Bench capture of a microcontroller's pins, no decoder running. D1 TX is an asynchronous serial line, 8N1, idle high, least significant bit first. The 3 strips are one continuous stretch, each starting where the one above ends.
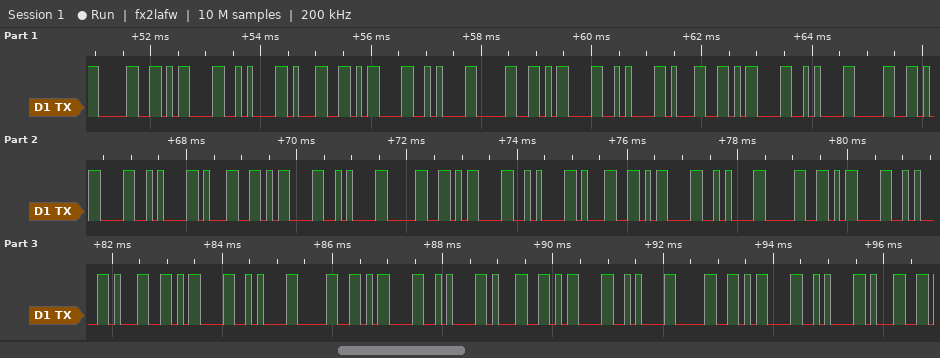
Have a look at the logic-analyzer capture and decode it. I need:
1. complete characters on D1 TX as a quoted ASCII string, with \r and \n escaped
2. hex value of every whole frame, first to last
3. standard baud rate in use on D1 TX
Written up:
"0\r\n1\r\n0\r\n1\r\n0\r\n1\r\n0\r\n1\r\n0\r\n1\r\n0\r\n1\r\n0\r\n1"
30 0D 0A 31 0D 0A 30 0D 0A 31 0D 0A 30 0D 0A 31 0D 0A 30 0D 0A 31 0D 0A 30 0D 0A 31 0D 0A 30 0D 0A 31 0D 0A 30 0D 0A 31
9600 baud
